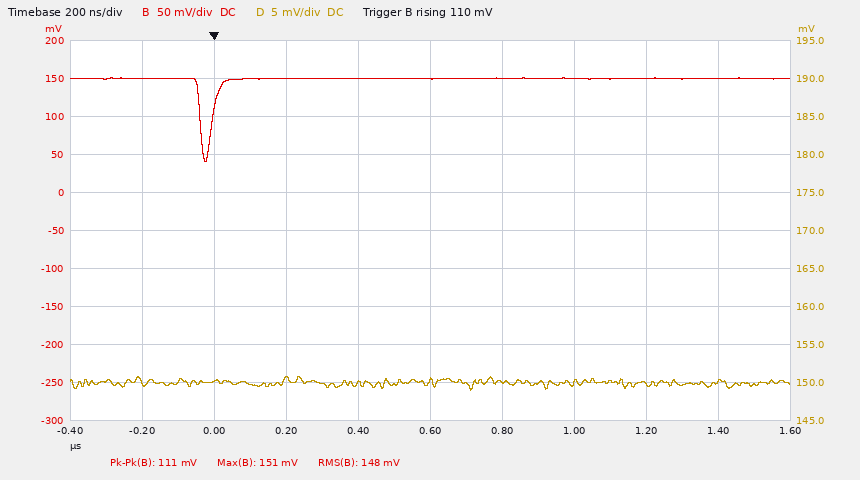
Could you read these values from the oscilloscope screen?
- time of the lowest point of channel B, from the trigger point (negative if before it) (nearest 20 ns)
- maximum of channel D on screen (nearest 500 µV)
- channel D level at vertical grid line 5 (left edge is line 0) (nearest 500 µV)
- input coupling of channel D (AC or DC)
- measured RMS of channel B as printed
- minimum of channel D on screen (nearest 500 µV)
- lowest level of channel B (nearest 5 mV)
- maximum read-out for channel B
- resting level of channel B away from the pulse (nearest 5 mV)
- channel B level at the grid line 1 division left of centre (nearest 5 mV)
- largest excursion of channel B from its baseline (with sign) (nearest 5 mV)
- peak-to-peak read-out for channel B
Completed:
-20 ns
151.0 mV
150.0 mV
DC
148 mV
149.0 mV
40 mV
151 mV
150 mV
150 mV
-110 mV
111 mV
